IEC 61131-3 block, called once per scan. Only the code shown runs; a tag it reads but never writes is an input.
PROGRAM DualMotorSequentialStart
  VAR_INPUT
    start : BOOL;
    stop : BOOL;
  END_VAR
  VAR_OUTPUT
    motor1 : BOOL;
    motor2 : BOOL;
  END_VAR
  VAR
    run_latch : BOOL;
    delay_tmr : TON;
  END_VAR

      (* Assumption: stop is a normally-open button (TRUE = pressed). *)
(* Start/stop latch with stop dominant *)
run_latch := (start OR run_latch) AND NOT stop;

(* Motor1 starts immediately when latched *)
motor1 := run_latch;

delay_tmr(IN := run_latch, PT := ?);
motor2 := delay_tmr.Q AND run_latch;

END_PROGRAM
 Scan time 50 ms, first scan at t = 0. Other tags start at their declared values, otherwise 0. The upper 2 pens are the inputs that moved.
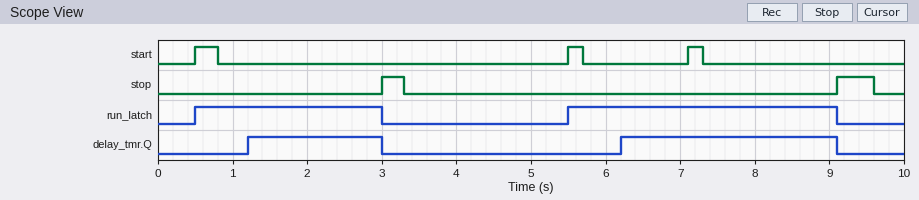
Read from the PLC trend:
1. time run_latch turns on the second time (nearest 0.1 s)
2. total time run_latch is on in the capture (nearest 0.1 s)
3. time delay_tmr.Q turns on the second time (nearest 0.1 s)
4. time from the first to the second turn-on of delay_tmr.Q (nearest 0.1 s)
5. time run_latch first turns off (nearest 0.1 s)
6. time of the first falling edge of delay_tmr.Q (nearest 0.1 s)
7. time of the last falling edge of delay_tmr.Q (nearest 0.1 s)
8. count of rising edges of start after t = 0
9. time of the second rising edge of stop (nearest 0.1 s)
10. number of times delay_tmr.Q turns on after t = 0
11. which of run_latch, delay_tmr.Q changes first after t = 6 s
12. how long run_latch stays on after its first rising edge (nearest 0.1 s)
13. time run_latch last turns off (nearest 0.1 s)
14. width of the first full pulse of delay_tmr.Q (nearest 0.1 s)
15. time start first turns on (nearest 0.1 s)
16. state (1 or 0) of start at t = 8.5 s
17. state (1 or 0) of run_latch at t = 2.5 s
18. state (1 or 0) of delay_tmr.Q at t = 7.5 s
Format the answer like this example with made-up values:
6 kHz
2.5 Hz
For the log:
5.5 s
6.1 s
6.2 s
5.0 s
3.0 s
3.0 s
9.1 s
3
9.1 s
2
delay_tmr.Q
2.5 s
9.1 s
1.8 s
0.5 s
0
1
1
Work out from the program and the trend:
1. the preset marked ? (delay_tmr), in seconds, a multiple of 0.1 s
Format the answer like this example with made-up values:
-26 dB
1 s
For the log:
0.7 s
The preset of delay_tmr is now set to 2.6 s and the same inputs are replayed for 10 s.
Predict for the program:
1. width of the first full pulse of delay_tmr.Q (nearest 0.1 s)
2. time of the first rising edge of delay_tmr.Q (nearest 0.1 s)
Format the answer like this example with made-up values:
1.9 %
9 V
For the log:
1.0 s
8.1 s
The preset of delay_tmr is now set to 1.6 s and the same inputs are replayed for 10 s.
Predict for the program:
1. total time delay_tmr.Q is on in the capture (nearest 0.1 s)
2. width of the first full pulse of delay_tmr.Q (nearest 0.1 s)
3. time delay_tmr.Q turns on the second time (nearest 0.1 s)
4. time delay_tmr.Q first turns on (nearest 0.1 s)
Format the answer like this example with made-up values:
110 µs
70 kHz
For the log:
2.9 s
0.9 s
7.1 s
2.1 s
